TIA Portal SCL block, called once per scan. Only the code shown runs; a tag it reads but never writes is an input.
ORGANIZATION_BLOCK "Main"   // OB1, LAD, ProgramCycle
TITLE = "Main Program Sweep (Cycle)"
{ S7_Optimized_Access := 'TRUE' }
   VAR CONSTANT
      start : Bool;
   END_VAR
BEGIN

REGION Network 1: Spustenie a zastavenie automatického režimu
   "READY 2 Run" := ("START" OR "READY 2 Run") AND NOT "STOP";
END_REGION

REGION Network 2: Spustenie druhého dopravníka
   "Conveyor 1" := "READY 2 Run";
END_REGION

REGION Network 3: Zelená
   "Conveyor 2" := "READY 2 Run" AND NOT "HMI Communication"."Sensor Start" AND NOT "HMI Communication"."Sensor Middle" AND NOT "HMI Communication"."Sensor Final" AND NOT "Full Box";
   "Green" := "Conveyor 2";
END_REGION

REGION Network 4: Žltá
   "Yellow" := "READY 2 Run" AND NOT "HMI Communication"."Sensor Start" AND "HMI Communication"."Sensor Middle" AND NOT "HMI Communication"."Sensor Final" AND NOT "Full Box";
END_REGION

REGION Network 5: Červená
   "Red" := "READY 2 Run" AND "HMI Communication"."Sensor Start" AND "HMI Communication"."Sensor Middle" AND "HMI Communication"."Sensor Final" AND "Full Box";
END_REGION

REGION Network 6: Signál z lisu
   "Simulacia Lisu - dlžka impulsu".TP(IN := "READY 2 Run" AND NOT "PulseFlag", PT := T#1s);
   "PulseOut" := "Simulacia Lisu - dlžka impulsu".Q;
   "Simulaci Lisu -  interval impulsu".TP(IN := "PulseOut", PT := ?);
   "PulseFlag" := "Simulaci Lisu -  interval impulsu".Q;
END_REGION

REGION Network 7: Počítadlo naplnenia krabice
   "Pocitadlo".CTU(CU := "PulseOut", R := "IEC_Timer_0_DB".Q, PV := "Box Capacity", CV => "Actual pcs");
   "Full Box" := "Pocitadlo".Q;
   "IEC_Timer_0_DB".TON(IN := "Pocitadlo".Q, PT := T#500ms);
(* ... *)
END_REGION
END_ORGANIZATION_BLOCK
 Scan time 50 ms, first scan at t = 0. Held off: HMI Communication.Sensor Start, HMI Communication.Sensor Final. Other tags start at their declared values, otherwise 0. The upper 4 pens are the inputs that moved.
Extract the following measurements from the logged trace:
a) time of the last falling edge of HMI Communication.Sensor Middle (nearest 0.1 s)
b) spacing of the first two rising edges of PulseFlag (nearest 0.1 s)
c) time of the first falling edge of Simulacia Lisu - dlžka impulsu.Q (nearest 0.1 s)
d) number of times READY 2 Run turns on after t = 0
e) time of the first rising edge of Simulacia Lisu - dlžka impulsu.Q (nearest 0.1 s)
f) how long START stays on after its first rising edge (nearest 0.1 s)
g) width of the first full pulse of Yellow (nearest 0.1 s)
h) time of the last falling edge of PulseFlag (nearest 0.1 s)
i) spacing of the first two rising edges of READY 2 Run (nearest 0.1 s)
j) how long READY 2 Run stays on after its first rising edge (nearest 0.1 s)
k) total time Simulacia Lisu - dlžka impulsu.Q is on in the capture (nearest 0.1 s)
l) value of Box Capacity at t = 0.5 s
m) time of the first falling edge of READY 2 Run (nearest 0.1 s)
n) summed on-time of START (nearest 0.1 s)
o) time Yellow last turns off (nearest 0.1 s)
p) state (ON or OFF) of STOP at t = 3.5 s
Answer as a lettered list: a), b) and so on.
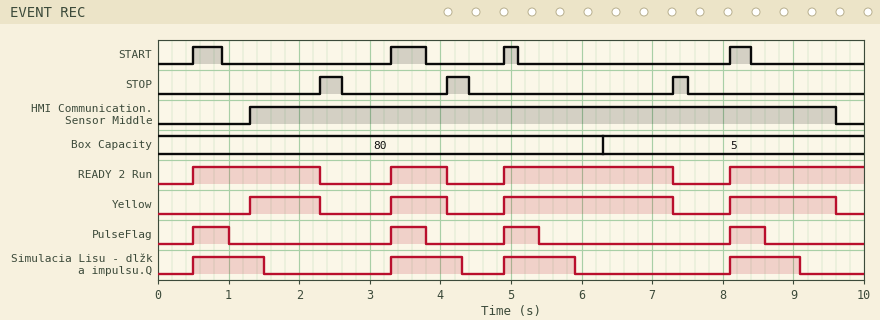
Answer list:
a) 9.6 s
b) 2.8 s
c) 1.5 s
d) 4
e) 0.5 s
f) 0.4 s
g) 1.0 s
h) 8.6 s
i) 2.8 s
j) 1.8 s
k) 4.0 s
l) 80
m) 2.3 s
n) 1.4 s
o) 9.6 s
p) OFF
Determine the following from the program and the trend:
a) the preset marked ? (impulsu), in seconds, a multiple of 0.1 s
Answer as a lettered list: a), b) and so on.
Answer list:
a) 0.5 s
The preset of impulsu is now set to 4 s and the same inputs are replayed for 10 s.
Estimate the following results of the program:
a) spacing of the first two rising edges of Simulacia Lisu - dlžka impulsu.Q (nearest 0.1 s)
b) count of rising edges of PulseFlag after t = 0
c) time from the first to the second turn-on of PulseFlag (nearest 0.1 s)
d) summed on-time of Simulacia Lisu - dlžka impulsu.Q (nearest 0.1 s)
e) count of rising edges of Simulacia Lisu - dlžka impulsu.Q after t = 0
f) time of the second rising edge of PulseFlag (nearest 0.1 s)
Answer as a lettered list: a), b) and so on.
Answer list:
a) 4.4 s
b) 3
c) 4.4 s
d) 3.0 s
e) 3
f) 4.9 s
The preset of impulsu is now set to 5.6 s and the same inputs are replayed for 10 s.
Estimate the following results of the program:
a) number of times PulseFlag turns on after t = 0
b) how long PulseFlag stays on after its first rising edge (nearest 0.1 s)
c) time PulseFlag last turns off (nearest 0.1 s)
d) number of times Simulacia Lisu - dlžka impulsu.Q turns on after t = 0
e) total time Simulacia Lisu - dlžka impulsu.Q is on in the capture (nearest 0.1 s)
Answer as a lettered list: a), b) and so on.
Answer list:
a) 2
b) 5.6 s
c) 6.1 s
d) 2
e) 2.0 s
